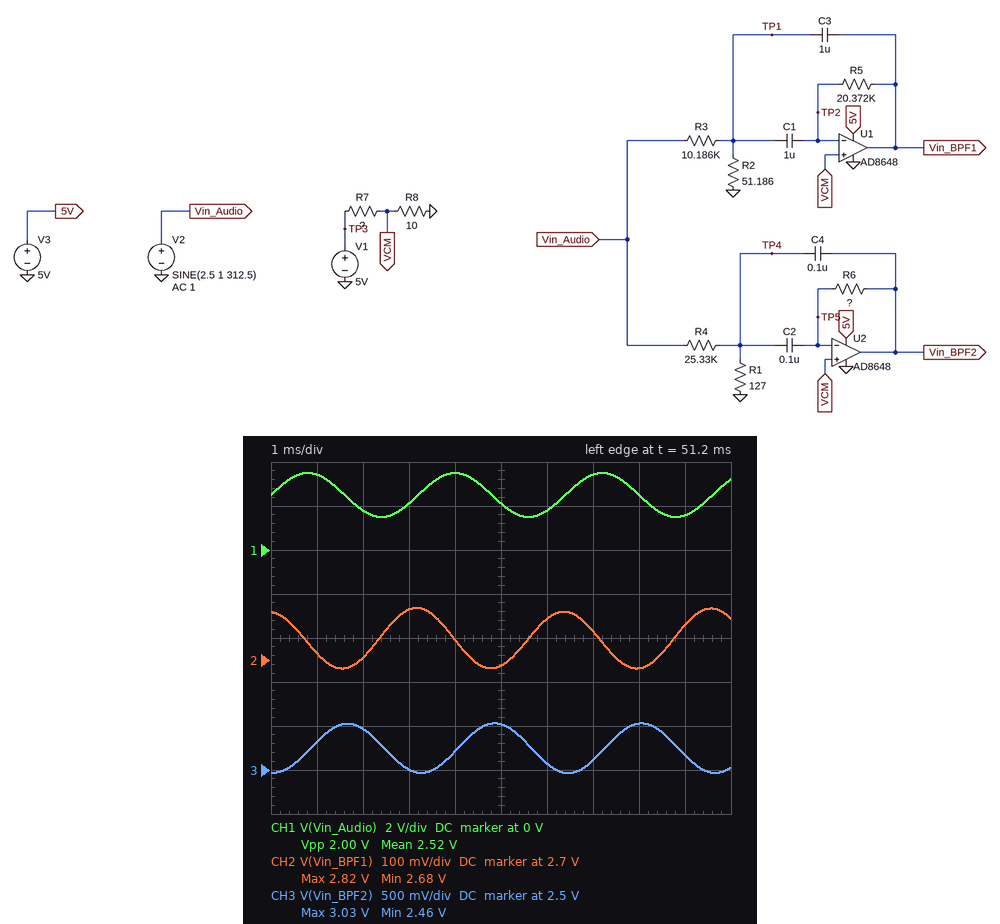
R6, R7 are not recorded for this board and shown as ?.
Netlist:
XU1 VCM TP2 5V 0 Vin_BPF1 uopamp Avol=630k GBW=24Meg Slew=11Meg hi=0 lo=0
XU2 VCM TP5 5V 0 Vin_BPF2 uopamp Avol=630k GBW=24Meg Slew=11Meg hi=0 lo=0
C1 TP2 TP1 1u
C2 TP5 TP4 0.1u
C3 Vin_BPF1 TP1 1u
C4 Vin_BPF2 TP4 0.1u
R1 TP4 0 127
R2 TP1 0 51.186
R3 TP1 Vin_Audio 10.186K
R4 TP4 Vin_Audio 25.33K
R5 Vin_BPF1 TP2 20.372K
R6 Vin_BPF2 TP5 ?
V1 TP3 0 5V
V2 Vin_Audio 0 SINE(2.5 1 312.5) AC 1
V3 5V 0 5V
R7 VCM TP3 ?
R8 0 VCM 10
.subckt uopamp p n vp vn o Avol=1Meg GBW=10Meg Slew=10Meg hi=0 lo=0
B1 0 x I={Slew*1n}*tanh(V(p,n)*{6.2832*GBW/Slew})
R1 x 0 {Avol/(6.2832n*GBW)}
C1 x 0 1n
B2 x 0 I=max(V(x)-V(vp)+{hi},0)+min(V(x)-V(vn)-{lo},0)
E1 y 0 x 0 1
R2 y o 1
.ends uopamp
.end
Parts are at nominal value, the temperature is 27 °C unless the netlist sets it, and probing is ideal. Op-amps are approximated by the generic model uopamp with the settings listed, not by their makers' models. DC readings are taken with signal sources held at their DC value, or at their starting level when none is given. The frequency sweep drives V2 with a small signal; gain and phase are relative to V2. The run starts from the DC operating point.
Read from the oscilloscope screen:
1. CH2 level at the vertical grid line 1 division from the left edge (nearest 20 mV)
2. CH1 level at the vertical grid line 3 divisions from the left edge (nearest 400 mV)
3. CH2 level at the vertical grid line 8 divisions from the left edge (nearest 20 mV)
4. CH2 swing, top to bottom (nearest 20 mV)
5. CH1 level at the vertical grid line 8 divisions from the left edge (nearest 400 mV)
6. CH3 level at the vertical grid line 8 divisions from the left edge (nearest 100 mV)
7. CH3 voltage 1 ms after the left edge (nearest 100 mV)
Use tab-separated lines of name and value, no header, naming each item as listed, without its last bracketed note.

CH2 level at the vertical grid line 1 division from the left edge	2.72 V
CH1 level at the vertical grid line 3 divisions from the left edge	2.0 V
CH2 level at the vertical grid line 8 divisions from the left edge	2.68 V
CH2 swing, top to bottom	140 mV
CH1 level at the vertical grid line 8 divisions from the left edge	2.4 V
CH3 level at the vertical grid line 8 divisions from the left edge	3.0 V
CH3 voltage 1 ms after the left edge	2.8 V
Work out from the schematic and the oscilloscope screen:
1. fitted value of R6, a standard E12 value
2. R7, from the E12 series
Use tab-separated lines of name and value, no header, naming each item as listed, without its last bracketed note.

fitted value of R6, a standard E12 value	120 kΩ
R7, from the E12 series	8.2 Ω
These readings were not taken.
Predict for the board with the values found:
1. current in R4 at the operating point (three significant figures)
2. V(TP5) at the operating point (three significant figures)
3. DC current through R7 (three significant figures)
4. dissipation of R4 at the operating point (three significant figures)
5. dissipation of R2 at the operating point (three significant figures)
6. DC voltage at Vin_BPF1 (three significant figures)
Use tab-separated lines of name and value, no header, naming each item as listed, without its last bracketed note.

current in R4 at the operating point	98.2 µA
V(TP5) at the operating point	2.75 V
DC current through R7	275 mA
dissipation of R4 at the operating point	244 µW
dissipation of R2 at the operating point	3.05 µW
DC voltage at Vin_BPF1	2.75 V
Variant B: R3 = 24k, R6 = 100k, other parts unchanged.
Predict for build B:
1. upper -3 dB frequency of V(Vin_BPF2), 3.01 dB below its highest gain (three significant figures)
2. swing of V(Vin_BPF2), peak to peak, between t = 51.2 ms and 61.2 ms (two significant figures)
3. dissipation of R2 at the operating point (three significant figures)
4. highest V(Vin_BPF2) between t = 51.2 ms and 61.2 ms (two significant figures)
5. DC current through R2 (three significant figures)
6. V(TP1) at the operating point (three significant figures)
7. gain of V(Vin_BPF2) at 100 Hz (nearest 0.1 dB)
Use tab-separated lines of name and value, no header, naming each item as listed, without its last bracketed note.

upper -3 dB frequency of V(Vin_BPF2), 3.01 dB below its highest gain	464 Hz
swing of V(Vin_BPF2), peak to peak, between t = 51.2 ms and 61.2 ms	380 mV
dissipation of R2 at the operating point	553 nW
highest V(Vin_BPF2) between t = 51.2 ms and 61.2 ms	2.9 V
DC current through R2	104 µA
V(TP1) at the operating point	5.32 mV
gain of V(Vin_BPF2) at 100 Hz	-29.6 dB
